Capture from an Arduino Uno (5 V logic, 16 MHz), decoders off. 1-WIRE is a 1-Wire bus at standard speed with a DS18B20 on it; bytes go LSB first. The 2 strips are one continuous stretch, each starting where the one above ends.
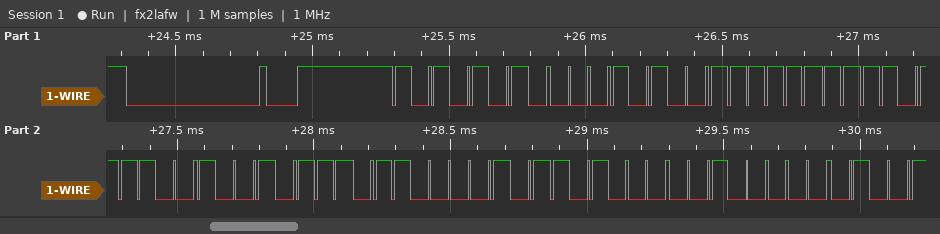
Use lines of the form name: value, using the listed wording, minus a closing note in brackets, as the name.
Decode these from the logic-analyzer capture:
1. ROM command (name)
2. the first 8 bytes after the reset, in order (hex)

ROM command: Match ROM
the first 8 bytes after the reset, in order: 55 28 FF 3B E9 86 16 04
